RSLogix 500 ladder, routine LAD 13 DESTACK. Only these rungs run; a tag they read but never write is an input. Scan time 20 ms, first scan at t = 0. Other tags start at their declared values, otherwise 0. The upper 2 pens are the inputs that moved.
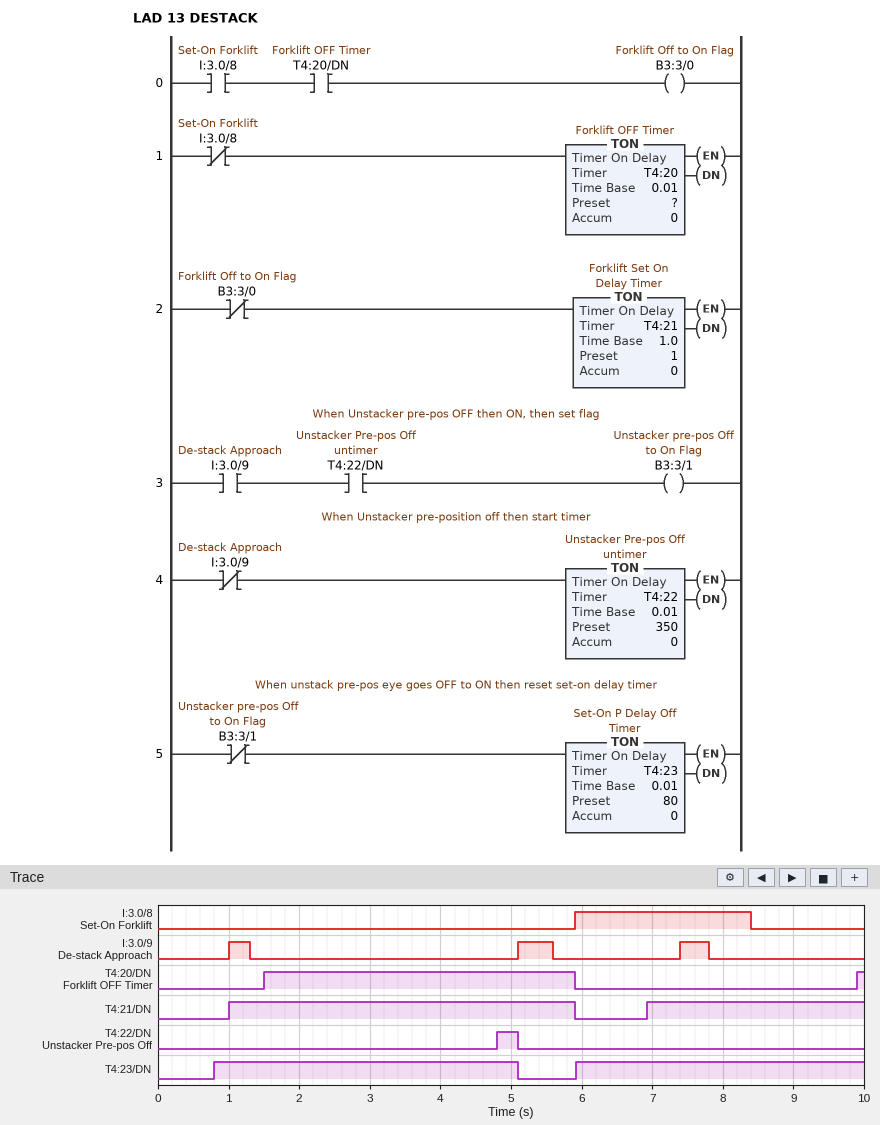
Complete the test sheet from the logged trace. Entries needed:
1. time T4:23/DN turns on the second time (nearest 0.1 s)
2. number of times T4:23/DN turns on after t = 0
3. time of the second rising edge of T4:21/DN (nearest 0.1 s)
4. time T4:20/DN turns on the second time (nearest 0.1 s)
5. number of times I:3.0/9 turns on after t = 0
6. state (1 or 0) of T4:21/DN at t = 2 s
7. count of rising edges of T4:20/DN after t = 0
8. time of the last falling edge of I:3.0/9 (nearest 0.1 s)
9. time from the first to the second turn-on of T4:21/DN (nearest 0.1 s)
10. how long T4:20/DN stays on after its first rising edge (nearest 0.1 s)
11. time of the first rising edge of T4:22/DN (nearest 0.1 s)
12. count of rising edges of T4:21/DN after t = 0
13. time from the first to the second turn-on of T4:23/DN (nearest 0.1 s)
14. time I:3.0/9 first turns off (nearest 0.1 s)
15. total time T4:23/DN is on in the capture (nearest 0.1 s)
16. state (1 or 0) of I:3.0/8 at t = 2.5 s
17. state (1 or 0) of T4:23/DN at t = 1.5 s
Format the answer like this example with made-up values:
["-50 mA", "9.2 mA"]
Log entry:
["5.9 s", "2", "6.9 s", "9.9 s", "3", "1", "2", "7.8 s", "5.9 s", "4.4 s", "4.8 s", "2", "5.1 s", "1.3 s", "8.4 s", "0", "1"]
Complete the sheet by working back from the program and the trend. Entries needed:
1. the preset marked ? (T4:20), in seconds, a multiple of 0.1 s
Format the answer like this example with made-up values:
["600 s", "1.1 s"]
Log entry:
["1.5 s"]
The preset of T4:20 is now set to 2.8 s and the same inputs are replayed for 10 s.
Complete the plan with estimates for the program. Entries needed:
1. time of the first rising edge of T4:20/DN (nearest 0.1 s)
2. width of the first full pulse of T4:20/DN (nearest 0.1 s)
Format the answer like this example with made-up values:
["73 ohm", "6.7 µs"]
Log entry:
["2.8 s", "3.1 s"]
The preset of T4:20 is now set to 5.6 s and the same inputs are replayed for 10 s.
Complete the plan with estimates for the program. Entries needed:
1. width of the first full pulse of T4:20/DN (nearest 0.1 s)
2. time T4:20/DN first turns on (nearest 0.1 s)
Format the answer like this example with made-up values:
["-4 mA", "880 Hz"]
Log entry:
["0.3 s", "5.6 s"]
